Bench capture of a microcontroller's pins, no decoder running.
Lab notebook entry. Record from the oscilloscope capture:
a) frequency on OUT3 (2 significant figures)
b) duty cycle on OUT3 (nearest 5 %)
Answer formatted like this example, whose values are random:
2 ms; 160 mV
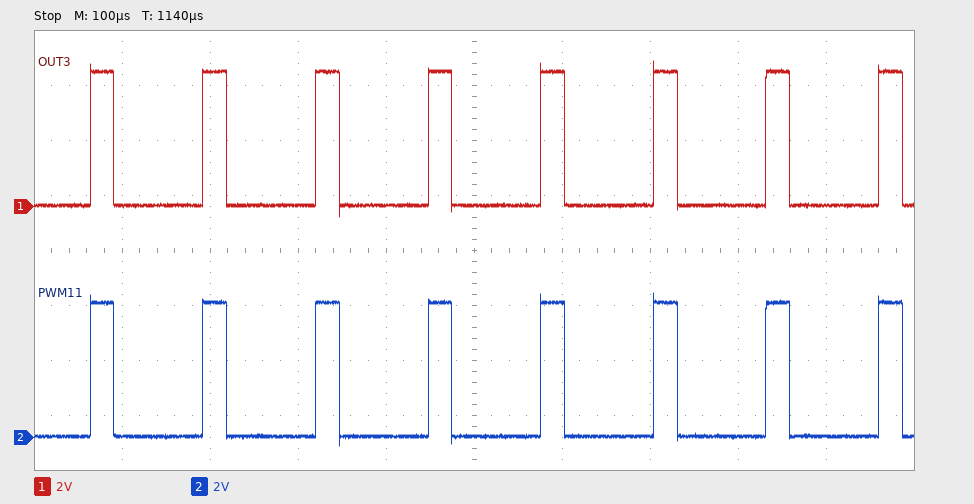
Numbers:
7.8 kHz; 20 %
